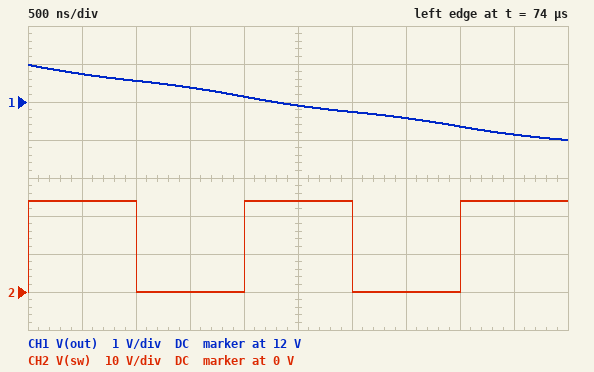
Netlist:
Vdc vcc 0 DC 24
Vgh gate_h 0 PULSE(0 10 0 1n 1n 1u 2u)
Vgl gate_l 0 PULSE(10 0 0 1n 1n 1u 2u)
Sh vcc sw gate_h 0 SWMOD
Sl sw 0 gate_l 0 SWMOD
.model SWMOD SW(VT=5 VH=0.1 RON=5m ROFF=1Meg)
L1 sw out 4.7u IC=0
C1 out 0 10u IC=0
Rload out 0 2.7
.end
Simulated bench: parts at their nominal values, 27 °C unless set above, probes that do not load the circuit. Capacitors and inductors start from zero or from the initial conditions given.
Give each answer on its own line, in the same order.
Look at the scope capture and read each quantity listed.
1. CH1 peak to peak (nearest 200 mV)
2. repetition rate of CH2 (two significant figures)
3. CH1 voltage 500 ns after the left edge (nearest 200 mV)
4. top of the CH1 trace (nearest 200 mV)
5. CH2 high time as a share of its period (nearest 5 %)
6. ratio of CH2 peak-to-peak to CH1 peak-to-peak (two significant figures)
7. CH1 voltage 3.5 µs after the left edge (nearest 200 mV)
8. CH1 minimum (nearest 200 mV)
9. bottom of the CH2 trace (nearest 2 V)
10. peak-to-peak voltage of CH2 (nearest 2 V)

2.0 V
500 kHz
12.8 V
13.0 V
50 %
12
11.6 V
11.0 V
0 V
24 V
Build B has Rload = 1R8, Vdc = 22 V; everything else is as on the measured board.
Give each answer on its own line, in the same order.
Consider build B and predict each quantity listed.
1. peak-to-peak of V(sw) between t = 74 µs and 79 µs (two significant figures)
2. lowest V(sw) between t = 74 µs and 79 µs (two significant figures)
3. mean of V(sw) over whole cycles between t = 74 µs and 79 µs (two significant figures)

22 V
-28 mV
11 V
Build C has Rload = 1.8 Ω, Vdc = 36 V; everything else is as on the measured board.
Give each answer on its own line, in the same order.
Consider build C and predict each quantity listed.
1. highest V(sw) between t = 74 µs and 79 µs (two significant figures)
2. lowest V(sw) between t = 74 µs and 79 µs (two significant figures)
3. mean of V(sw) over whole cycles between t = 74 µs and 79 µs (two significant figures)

36 V
-46 mV
18 V
